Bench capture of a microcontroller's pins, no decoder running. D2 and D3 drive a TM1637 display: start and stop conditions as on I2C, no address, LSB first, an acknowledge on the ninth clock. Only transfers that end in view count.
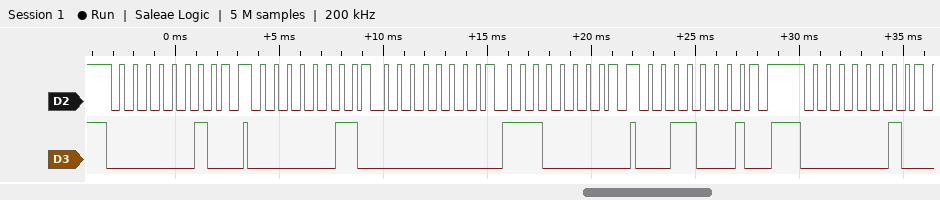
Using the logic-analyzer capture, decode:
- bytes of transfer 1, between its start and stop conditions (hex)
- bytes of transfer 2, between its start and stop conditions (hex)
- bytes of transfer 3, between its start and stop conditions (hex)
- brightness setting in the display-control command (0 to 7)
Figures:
40
C0 00 07
8C
4
